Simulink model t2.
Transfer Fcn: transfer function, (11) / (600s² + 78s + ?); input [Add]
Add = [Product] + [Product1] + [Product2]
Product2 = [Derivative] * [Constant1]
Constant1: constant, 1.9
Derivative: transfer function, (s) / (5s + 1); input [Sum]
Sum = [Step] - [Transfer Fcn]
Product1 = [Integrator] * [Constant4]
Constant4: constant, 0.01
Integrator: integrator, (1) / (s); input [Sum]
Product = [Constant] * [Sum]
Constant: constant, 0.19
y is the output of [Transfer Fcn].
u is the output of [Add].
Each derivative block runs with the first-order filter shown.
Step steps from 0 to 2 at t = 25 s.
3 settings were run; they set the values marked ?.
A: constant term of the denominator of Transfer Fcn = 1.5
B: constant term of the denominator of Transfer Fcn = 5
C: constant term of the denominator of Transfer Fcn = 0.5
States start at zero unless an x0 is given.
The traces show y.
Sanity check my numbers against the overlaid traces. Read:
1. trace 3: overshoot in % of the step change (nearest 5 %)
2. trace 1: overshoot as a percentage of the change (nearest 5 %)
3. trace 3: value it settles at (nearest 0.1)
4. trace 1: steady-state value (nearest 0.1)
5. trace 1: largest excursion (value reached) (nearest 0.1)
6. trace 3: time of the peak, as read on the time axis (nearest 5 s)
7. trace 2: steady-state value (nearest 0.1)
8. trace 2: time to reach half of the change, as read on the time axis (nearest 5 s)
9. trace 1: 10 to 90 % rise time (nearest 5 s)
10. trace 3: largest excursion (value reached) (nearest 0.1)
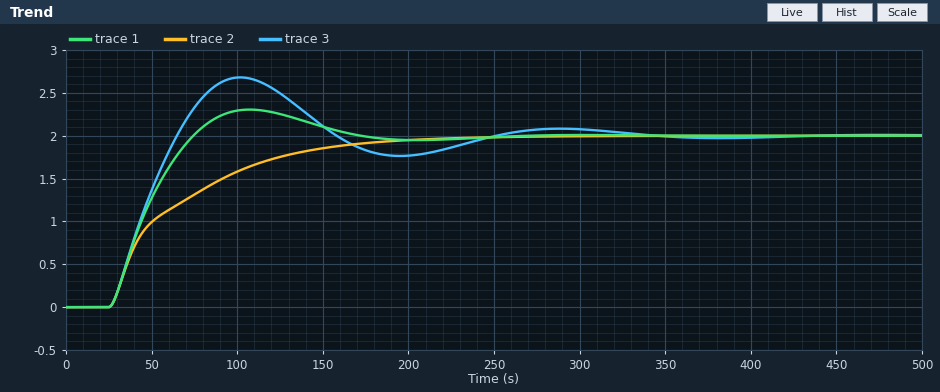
35 %
15 %
2.0
2.0
2.3
100 s
2.0
50 s
35 s
2.7
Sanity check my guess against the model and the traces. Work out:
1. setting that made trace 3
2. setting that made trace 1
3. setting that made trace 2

C
A
B
